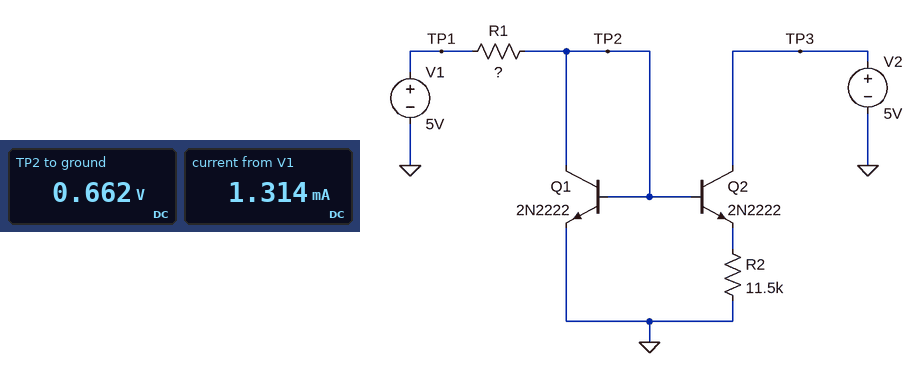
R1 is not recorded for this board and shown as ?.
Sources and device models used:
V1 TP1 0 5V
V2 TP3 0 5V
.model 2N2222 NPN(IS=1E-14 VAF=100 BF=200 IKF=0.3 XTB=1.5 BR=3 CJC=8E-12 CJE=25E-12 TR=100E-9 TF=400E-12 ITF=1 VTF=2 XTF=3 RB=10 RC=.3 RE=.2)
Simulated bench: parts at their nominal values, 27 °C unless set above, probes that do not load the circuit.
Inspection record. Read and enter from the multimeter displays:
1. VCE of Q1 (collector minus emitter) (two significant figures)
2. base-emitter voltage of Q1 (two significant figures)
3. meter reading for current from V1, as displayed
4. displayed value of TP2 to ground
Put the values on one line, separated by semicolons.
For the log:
660 mV; 660 mV; 1.314 mA; 0.662 V
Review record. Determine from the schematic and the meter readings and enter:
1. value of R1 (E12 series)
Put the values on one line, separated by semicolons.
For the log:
3.3 kΩ
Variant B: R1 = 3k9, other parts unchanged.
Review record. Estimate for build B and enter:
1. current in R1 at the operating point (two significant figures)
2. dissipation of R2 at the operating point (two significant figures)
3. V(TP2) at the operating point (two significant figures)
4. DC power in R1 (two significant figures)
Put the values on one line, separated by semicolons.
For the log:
1.1 mA; 1.3 µW; 660 mV; 4.8 mW
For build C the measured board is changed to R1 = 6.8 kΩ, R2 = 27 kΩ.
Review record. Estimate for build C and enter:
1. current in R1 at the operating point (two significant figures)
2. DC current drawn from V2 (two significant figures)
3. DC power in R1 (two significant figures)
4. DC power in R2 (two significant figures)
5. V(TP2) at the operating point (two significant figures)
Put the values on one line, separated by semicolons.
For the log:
640 µA; 4.7 µA; 2.8 mW; 610 nW; 640 mV
